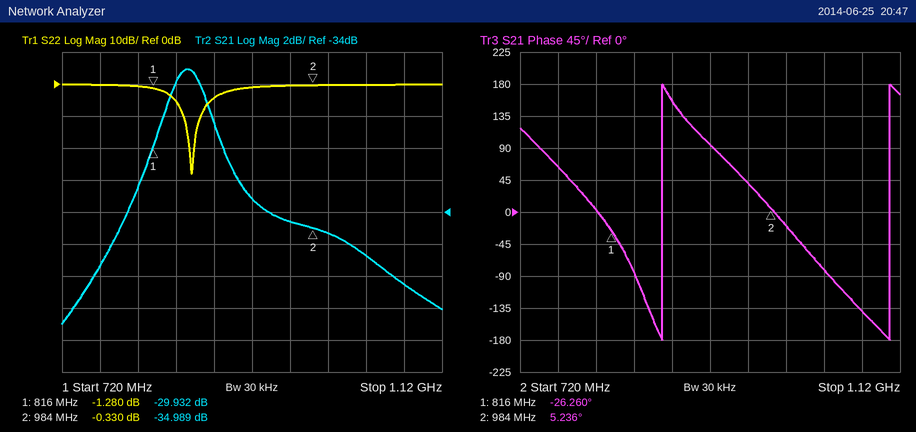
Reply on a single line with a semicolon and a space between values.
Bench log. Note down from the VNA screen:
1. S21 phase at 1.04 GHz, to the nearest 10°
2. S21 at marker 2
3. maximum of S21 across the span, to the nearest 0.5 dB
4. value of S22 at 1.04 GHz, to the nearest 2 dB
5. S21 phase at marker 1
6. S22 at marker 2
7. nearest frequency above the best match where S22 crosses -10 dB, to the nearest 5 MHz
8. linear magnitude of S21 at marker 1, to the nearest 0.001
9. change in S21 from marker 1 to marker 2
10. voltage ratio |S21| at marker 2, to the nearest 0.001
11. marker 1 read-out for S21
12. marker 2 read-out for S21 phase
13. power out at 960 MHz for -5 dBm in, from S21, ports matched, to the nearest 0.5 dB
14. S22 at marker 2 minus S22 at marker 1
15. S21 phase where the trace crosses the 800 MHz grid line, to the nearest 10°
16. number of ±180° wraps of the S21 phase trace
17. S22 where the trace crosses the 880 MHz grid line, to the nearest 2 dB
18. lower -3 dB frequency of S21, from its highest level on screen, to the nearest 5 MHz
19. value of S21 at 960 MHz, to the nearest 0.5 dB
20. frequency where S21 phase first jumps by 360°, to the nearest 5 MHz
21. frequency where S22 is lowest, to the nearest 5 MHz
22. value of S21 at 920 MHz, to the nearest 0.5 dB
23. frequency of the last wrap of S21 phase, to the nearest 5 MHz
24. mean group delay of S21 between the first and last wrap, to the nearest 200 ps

-80°; -34.989 dB; -25.0 dB; 0 dB; -26.260°; -0.330 dB; 865 MHz; 0.032; -5.057 dB; 0.018; -29.932 dB; 5.236°; -39.5 dBm; 0.950 dB; 0°; 2; -4 dB; 825 MHz; -34.5 dB; 870 MHz; 855 MHz; -33.0 dB; 1.110 GHz; 4.2 ns
